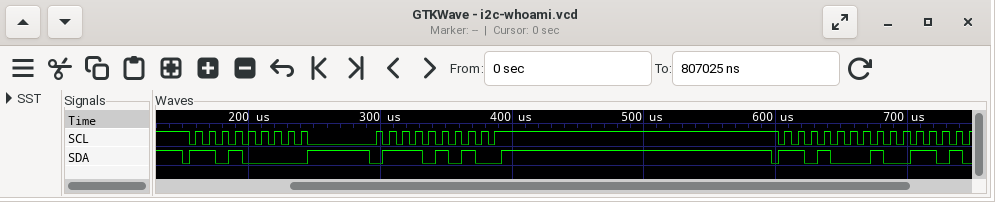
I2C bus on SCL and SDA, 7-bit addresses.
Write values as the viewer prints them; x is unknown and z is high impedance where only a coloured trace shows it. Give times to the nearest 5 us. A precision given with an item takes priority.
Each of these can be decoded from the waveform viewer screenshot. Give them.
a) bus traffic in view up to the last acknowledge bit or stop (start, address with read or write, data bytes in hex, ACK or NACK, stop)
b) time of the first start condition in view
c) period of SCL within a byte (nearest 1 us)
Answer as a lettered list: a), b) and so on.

a) start, address 68 write ACK, 75 ACK, stop, start, address 68 read ACK
b) 150 us
c) 10 us
